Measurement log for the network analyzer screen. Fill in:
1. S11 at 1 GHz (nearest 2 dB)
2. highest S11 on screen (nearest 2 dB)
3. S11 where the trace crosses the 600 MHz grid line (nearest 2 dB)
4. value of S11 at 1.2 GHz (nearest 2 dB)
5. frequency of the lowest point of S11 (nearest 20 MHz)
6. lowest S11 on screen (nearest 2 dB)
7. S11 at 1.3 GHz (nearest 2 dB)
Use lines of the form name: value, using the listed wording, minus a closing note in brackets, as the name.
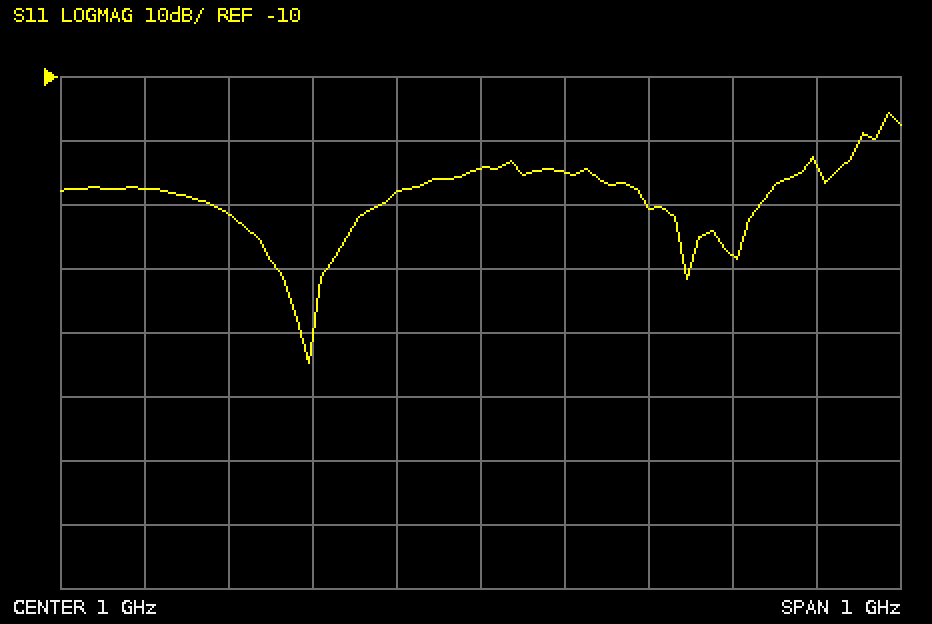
S11 at 1 GHz: -24 dB
highest S11 on screen: -16 dB
S11 where the trace crosses the 600 MHz grid line: -28 dB
value of S11 at 1.2 GHz: -30 dB
frequency of the lowest point of S11: 800 MHz
lowest S11 on screen: -54 dB
S11 at 1.3 GHz: -38 dB
